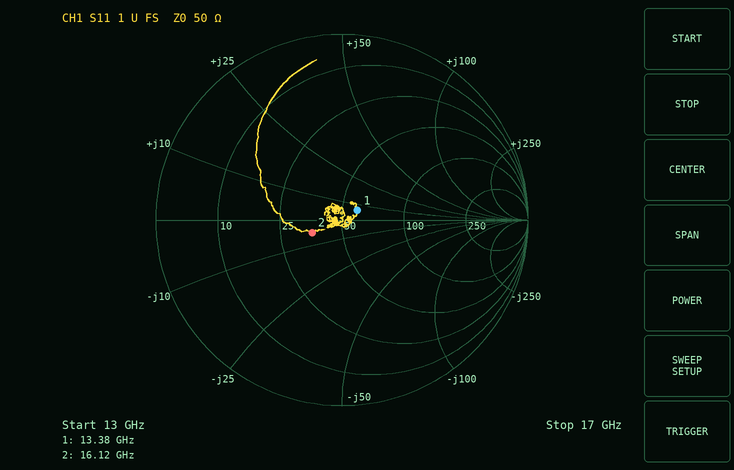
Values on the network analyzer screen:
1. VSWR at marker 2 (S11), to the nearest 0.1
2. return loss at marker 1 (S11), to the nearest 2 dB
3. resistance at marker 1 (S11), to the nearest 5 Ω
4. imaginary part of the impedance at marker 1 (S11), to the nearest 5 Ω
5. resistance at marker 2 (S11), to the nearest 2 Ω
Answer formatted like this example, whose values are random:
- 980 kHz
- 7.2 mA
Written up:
- 1.4
- 20 dB
- 60 Ω
- +5 Ω
- 36 Ω
